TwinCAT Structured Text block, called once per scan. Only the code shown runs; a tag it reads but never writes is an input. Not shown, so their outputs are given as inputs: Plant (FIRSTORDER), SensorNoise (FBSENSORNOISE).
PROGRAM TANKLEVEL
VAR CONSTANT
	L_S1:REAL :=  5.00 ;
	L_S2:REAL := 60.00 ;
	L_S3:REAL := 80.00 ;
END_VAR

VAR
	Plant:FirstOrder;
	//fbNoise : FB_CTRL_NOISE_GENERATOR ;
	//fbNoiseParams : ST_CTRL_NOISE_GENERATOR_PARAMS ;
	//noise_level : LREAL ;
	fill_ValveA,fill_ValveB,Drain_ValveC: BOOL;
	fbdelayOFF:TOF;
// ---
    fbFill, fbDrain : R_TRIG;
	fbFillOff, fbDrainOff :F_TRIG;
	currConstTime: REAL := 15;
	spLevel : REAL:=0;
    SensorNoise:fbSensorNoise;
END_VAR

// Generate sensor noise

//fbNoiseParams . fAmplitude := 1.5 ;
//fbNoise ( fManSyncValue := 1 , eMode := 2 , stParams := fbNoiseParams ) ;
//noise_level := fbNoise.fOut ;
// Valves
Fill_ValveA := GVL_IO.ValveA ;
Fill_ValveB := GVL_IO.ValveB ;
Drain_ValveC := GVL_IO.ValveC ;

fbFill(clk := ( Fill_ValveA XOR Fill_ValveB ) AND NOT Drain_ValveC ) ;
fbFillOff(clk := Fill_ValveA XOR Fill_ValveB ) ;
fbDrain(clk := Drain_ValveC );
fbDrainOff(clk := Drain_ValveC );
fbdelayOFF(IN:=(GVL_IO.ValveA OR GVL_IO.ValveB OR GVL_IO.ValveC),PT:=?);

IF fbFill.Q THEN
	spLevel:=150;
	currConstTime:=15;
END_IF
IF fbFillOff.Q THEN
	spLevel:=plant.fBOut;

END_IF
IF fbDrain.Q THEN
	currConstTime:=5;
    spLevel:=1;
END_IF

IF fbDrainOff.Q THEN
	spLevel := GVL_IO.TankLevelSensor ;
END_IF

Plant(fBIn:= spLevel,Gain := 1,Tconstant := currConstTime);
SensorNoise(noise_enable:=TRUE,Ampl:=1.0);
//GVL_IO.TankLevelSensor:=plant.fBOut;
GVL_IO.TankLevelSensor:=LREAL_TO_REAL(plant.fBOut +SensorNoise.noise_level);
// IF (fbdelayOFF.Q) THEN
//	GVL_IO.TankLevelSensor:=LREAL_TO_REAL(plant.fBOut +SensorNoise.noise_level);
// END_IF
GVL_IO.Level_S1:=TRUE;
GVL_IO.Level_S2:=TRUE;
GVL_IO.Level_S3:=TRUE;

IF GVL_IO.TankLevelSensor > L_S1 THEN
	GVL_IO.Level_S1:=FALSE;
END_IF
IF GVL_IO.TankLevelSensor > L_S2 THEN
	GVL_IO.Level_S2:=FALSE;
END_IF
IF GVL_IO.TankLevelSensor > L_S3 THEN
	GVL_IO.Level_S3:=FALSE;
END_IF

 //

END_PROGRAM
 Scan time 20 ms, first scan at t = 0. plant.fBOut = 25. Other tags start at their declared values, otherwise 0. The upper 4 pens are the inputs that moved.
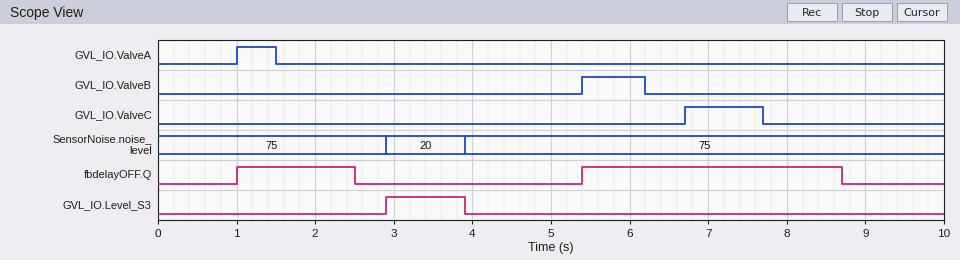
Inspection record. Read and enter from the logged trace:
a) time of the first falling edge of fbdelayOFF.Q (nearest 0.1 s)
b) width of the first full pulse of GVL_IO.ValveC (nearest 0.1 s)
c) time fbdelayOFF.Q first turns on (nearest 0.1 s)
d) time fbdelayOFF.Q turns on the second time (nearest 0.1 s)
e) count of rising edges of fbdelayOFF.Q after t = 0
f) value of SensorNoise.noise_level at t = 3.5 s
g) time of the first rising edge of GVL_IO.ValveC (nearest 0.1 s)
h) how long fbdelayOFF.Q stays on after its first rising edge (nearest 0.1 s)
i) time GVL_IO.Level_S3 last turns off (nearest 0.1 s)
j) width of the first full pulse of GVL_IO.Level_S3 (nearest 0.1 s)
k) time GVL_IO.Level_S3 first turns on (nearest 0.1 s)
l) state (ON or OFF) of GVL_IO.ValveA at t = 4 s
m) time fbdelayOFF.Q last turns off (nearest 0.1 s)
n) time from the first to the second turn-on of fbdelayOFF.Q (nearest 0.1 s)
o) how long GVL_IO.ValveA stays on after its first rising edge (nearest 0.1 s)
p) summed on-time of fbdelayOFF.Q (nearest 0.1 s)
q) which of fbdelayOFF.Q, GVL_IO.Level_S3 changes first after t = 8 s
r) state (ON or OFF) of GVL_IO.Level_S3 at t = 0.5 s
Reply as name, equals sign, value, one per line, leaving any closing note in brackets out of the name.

time of the first falling edge of fbdelayOFF.Q = 2.5 s
width of the first full pulse of GVL_IO.ValveC = 1.0 s
time fbdelayOFF.Q first turns on = 1.0 s
time fbdelayOFF.Q turns on the second time = 5.4 s
count of rising edges of fbdelayOFF.Q after t = 0 = 2
value of SensorNoise.noise_level at t = 3.5 s = 20
time of the first rising edge of GVL_IO.ValveC = 6.7 s
how long fbdelayOFF.Q stays on after its first rising edge = 1.5 s
time GVL_IO.Level_S3 last turns off = 3.9 s
width of the first full pulse of GVL_IO.Level_S3 = 1.0 s
time GVL_IO.Level_S3 first turns on = 2.9 s
state (ON or OFF) of GVL_IO.ValveA at t = 4 s = OFF
time fbdelayOFF.Q last turns off = 8.7 s
time from the first to the second turn-on of fbdelayOFF.Q = 4.4 s
how long GVL_IO.ValveA stays on after its first rising edge = 0.5 s
summed on-time of fbdelayOFF.Q = 4.8 s
which of fbdelayOFF.Q, GVL_IO.Level_S3 changes first after t = 8 s = fbdelayOFF.Q
state (ON or OFF) of GVL_IO.Level_S3 at t = 0.5 s = OFF
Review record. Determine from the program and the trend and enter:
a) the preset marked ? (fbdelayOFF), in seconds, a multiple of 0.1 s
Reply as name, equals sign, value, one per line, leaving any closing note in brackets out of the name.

the preset marked ? (fbdelayOFF), in seconds, a multiple of 0.1 s = 1.0 s
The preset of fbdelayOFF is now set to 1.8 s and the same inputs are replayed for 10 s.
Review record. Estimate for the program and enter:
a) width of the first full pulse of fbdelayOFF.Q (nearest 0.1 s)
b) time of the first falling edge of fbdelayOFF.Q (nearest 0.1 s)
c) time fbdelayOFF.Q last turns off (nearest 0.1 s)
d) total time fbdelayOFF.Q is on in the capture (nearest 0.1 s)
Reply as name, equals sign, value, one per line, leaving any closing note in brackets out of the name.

width of the first full pulse of fbdelayOFF.Q = 2.3 s
time of the first falling edge of fbdelayOFF.Q = 3.3 s
time fbdelayOFF.Q last turns off = 9.5 s
total time fbdelayOFF.Q is on in the capture = 6.4 s
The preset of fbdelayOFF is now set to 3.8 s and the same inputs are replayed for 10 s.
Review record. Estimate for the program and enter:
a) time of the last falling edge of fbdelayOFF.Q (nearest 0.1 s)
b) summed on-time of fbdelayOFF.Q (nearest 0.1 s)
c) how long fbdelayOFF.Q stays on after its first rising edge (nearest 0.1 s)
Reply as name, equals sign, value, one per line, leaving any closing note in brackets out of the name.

time of the last falling edge of fbdelayOFF.Q = 5.3 s
summed on-time of fbdelayOFF.Q = 8.9 s
how long fbdelayOFF.Q stays on after its first rising edge = 4.3 s
